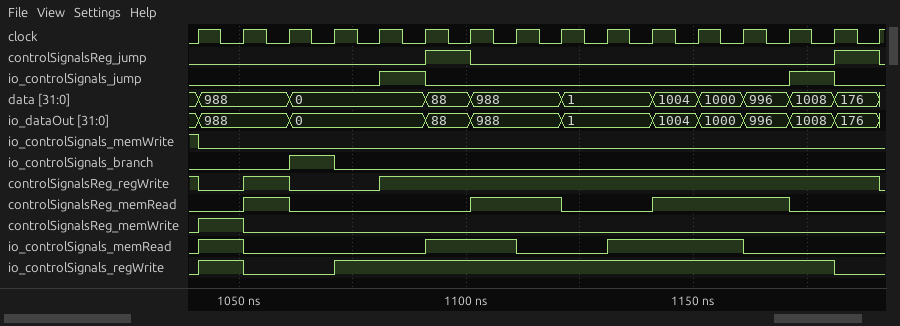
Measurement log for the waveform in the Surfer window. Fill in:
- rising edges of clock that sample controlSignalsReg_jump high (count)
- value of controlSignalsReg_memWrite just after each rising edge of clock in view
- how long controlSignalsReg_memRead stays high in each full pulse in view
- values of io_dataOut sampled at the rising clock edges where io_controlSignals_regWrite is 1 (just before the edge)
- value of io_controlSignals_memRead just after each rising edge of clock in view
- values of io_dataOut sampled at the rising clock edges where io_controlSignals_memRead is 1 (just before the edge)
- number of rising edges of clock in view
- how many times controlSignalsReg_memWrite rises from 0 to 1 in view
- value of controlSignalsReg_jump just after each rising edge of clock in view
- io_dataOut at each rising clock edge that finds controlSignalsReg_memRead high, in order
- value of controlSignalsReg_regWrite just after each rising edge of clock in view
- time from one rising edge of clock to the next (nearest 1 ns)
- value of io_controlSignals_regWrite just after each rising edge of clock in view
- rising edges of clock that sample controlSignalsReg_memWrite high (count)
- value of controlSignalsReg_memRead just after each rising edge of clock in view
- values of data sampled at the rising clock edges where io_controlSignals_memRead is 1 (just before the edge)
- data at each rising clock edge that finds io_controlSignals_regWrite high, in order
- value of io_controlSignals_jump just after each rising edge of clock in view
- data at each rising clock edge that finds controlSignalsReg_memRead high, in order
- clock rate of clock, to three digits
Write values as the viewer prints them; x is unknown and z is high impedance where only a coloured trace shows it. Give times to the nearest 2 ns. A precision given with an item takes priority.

2
1 0 0 0 0 0 0 0 0 0 0 0 0 0 0 0
10 ns, 20 ns, 30 ns
988, 0, 0, 88, 988, 988, 1, 1, 1004, 1000, 996, 1008
1 0 0 0 0 1 1 0 0 1 1 1 0 0 0 0
988, 88, 988, 1, 1004, 1000
16
1
0 0 0 0 0 1 0 0 0 0 0 0 0 0 1 0
988, 988, 988, 1004, 1000, 996
0 1 0 0 1 1 1 1 1 1 1 1 1 1 1 0
10 ns
1 0 0 1 1 1 1 1 1 1 1 1 1 1 0 0
1
0 1 0 0 0 0 1 1 0 0 1 1 1 0 0 0
988, 88, 988, 1, 1004, 1000
988, 0, 0, 88, 988, 988, 1, 1, 1004, 1000, 996, 1008
0 0 0 0 1 0 0 0 0 0 0 0 0 1 0 0
988, 988, 988, 1004, 1000, 996
100 MHz
